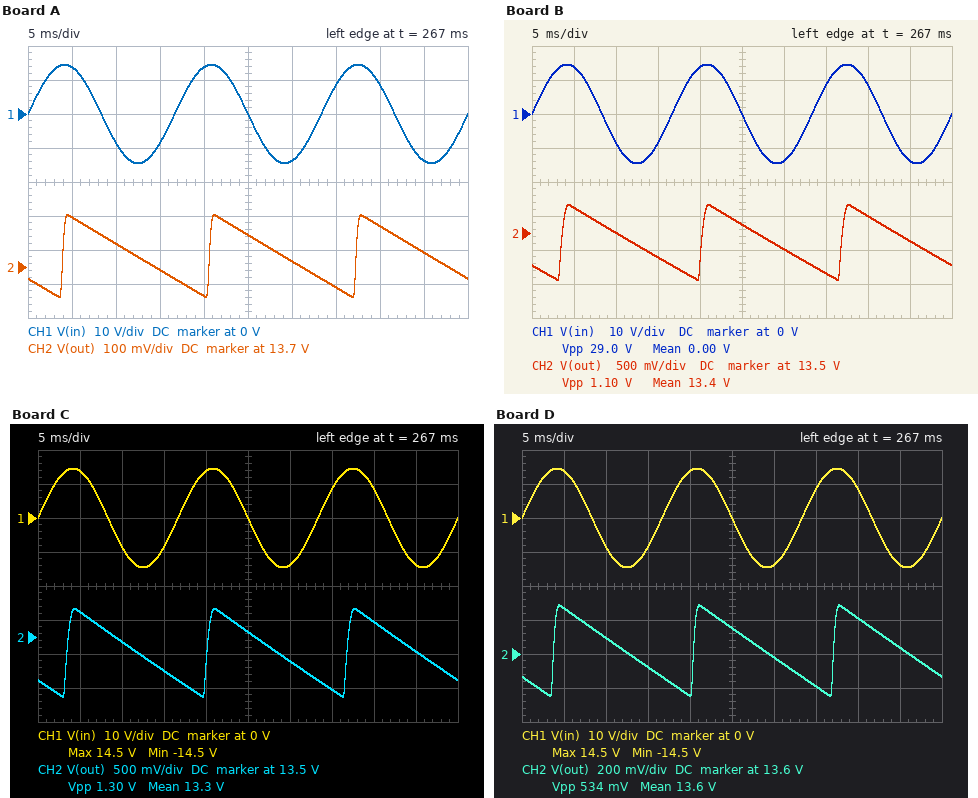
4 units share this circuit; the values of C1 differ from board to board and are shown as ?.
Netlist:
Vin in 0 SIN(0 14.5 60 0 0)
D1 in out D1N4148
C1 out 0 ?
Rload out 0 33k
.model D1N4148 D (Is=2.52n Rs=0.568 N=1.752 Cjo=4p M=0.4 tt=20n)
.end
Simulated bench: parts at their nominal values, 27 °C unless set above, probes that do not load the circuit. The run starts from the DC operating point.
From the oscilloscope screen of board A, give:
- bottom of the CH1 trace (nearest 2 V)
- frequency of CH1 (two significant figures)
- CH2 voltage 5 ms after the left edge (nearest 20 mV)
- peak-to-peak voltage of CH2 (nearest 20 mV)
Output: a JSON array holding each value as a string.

["-14 V", "60 Hz", "13.84 V", "240 mV"]
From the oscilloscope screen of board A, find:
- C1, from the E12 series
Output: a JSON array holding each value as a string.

["27 µF"]
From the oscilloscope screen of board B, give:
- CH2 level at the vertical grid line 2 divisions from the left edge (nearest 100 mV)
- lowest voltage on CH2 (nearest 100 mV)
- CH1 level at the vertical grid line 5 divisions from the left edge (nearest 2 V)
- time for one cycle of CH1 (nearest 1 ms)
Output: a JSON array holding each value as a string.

["13.5 V", "12.8 V", "0 V", "17 ms"]
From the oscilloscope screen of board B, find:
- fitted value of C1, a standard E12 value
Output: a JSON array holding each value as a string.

["5.6 µF"]
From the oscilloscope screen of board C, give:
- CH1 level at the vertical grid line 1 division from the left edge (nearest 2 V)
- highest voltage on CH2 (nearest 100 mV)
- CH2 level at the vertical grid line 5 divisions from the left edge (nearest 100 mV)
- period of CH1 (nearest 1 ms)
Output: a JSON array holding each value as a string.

["14 V", "13.9 V", "13.6 V", "17 ms"]
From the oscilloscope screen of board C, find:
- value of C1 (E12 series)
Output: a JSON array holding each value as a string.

["4.7 µF"]
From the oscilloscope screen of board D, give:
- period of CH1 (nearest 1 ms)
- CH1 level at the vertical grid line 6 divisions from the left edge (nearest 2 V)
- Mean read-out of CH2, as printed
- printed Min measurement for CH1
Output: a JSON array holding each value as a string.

["17 ms", "-14 V", "13.6 V", "-14.5 V"]
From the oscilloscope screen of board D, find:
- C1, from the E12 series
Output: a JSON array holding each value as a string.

["12 µF"]
